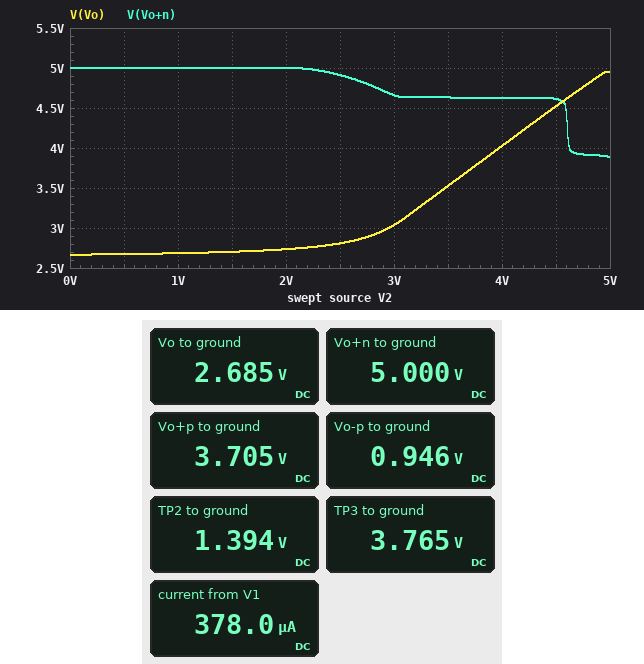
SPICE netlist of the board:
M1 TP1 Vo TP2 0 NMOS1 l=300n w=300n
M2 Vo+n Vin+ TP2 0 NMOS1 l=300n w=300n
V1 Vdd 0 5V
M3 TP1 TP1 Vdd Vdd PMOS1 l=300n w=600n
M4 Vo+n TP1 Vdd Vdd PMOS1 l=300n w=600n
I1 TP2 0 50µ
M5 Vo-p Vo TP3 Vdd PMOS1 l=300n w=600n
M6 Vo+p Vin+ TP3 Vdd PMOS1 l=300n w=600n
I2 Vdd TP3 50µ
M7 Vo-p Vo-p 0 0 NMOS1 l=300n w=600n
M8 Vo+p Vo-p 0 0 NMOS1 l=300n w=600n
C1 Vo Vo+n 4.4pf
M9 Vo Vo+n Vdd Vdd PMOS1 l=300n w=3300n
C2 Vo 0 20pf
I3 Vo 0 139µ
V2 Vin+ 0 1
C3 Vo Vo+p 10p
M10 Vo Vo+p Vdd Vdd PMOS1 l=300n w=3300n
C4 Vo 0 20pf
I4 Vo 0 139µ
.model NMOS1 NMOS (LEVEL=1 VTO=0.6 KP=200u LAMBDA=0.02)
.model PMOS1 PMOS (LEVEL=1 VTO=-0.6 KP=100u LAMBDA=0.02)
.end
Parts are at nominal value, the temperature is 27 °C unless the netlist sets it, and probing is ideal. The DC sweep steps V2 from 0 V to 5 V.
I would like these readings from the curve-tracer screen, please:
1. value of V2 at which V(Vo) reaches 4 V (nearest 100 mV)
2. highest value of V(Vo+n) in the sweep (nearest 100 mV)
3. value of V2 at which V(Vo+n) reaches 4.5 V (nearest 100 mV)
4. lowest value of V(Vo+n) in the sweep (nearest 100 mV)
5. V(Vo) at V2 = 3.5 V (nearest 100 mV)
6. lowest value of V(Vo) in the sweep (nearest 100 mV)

4.0 V
5.0 V
4.6 V
3.9 V
3.5 V
2.7 V
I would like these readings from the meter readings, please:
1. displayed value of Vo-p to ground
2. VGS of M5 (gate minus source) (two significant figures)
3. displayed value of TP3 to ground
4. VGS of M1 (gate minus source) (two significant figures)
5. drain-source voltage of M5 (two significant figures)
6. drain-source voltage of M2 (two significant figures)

0.946 V
-1.1 V
3.765 V
1.3 V
-2.8 V
3.6 V
